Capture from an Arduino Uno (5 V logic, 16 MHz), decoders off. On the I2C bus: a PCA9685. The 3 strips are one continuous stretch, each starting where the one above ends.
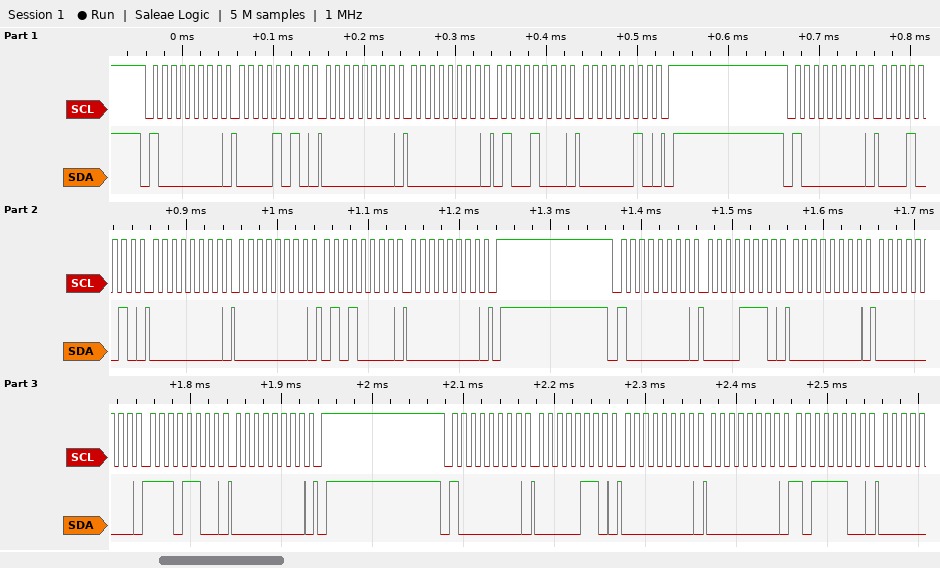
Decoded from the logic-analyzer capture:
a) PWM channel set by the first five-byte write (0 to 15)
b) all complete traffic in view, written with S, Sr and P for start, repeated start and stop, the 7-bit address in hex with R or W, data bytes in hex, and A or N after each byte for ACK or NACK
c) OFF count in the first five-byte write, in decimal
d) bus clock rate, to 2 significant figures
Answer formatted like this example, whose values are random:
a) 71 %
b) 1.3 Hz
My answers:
a) 1
b) S 40W A 0A A 00 A 00 A 48 A 02 A P S 40W A 12 A 00 A 00 A 50 A 00 A P S 40W A 0E A 00 A 00 A EC A 00 A P S 40W A 06 A 00 A 00 A BC A
c) 584
d) 100 kHz
